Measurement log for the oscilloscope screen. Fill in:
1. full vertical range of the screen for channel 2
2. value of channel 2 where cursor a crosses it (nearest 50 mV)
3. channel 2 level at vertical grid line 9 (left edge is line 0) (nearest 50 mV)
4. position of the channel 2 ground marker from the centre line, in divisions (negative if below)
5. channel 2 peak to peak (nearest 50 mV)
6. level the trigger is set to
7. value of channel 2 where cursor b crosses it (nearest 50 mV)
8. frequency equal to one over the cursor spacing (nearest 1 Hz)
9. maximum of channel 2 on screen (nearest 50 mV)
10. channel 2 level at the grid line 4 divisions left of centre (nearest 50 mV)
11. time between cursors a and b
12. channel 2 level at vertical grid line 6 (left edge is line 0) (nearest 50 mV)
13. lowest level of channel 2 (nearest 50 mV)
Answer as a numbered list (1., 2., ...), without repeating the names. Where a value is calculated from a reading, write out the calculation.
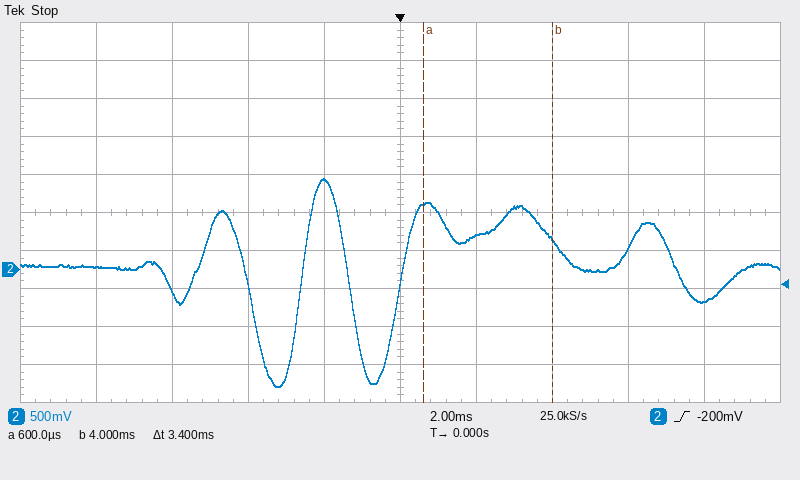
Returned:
1. 5 V
2. 850 mV
3. -400 mV
4. -1.5 div
5. 1.20 V − (-1.55 V) = 2.75 V
6. -200 mV
7. 400 mV
8. 1 / 3.4 ms ≈ 294 Hz
9. 1.20 V
10. 50 mV
11. 3.4 ms
12. 450 mV
13. -1.55 V
